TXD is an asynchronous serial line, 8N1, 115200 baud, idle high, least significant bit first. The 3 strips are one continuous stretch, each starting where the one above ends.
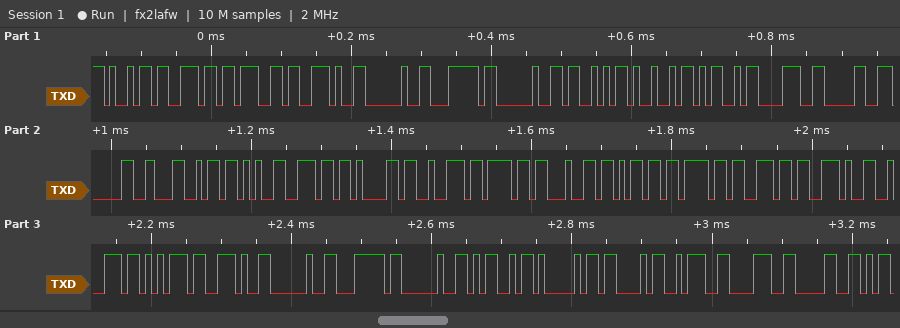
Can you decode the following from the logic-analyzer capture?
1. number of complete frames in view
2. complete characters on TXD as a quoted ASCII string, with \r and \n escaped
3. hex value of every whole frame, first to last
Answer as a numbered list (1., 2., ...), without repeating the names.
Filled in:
1. 36
2. "ing. | SIM800L+narodmon.ru. | MAC:80"
3. 69 6E 67 2E 20 7C 20 53 49 4D 38 30 30 4C 2B 6E 61 72 6F 64 6D 6F 6E 2E 72 75 2E 20 7C 20 4D 41 43 3A 38 30
